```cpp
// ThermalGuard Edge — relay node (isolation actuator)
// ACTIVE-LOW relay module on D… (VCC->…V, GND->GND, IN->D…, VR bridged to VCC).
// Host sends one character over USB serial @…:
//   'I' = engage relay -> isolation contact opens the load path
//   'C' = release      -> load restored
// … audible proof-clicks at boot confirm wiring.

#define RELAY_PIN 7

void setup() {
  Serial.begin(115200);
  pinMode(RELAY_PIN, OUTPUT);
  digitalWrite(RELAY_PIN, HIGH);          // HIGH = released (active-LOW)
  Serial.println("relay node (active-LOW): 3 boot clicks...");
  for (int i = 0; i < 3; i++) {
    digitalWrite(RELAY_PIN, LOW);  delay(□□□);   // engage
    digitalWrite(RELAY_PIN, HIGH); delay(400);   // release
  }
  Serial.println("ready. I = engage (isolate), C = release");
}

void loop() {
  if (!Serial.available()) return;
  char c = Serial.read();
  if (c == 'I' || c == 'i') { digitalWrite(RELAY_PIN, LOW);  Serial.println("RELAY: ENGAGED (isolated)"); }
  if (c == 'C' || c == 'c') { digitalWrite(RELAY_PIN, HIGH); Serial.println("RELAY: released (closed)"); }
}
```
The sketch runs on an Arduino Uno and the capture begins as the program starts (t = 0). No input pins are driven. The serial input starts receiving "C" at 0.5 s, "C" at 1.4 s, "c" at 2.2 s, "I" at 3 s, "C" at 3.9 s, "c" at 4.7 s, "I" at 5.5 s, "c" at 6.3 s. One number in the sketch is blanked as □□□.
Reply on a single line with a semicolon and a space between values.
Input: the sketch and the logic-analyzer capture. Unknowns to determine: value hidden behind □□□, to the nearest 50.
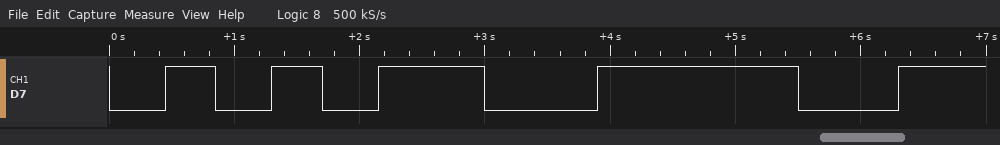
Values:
450
